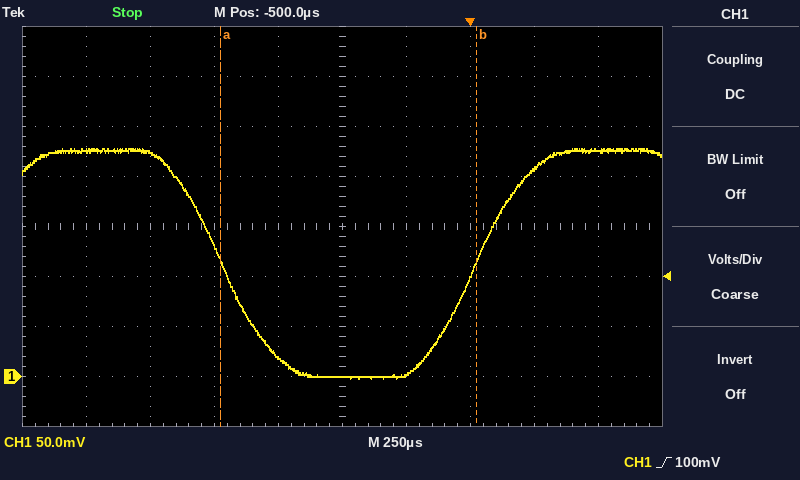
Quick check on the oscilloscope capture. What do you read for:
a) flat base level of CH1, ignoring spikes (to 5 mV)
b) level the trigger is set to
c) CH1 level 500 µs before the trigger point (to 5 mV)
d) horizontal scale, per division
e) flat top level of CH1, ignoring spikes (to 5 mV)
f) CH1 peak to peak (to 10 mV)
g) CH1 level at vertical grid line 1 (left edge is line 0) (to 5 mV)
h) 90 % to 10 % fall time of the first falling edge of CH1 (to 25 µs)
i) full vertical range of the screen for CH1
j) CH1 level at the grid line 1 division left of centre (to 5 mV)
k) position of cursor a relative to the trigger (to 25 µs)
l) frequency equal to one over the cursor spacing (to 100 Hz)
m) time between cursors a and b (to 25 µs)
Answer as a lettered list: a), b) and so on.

a) 0 mV
b) 100 mV
c) 0 mV
d) 250 µs
e) 225 mV
f) 230 mV
g) 225 mV
h) 400 µs
i) 400 mV
j) 20 mV
k) -975 µs
l) 1.0 kHz
m) 1.000 ms
